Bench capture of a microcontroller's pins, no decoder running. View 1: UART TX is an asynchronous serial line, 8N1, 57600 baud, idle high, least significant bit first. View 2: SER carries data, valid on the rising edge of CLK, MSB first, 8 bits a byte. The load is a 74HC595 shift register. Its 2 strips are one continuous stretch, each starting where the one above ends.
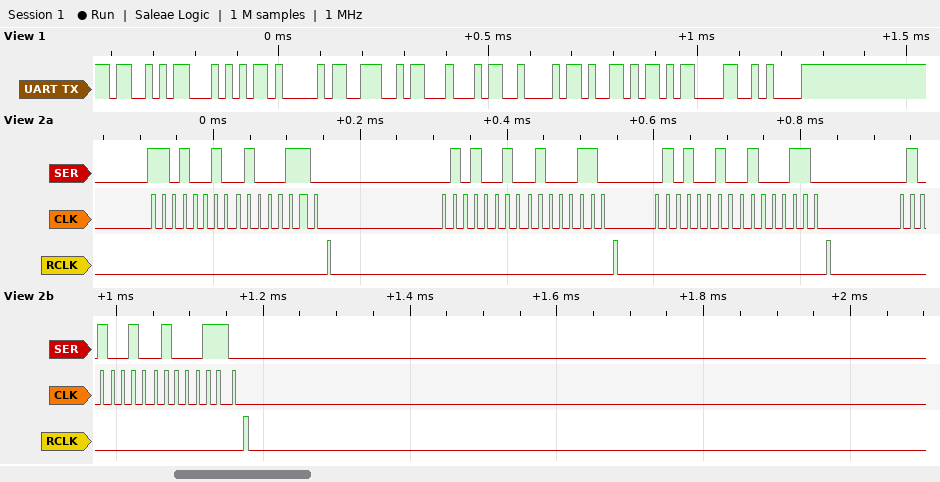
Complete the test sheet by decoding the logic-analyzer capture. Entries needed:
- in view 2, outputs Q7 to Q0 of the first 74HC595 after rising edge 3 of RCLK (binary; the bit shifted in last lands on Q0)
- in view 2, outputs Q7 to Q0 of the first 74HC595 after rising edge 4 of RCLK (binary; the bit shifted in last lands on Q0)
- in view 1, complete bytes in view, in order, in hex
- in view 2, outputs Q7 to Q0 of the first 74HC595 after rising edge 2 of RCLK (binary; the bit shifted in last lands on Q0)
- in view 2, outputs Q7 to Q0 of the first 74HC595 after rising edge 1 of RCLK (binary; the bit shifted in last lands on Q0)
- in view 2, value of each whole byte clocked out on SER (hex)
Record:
01000110
01000110
53 54 41 4E 44 42 59 0D 0A
01000110
01000110
0xD2 0x46 0x52 0x46 0x52 0x46 0x52 0x46
